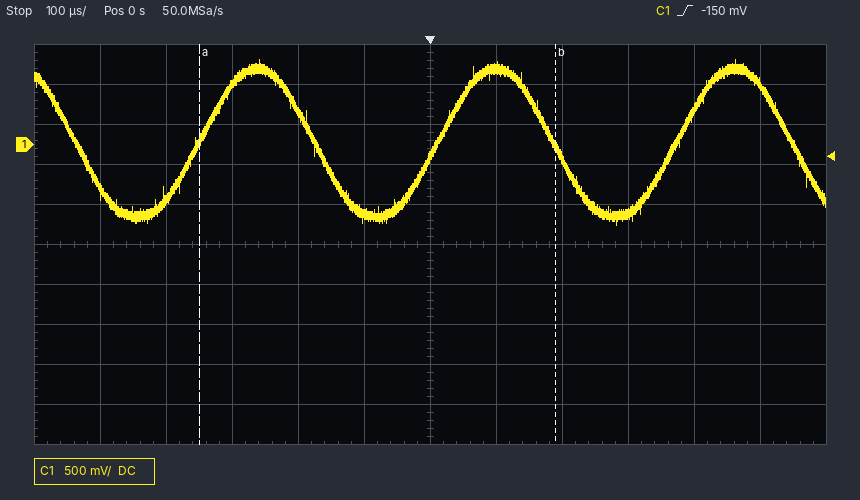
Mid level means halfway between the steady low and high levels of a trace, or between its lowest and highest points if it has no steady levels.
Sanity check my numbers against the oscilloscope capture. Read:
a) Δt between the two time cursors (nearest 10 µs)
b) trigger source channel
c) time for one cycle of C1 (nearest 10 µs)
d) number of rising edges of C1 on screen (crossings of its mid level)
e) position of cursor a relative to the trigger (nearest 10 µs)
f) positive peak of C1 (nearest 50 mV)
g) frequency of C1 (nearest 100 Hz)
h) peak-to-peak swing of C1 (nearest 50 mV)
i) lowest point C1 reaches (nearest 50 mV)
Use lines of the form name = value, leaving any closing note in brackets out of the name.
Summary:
Δt between the two time cursors = 540 µs
trigger source channel = C1
time for one cycle of C1 = 360 µs
number of rising edges of C1 on screen = 3
position of cursor a relative to the trigger = -350 µs
positive peak of C1 = 1.05 V
frequency of C1 = 2.8 kHz
peak-to-peak swing of C1 = 2.05 V
lowest point C1 reaches = -1.00 V
